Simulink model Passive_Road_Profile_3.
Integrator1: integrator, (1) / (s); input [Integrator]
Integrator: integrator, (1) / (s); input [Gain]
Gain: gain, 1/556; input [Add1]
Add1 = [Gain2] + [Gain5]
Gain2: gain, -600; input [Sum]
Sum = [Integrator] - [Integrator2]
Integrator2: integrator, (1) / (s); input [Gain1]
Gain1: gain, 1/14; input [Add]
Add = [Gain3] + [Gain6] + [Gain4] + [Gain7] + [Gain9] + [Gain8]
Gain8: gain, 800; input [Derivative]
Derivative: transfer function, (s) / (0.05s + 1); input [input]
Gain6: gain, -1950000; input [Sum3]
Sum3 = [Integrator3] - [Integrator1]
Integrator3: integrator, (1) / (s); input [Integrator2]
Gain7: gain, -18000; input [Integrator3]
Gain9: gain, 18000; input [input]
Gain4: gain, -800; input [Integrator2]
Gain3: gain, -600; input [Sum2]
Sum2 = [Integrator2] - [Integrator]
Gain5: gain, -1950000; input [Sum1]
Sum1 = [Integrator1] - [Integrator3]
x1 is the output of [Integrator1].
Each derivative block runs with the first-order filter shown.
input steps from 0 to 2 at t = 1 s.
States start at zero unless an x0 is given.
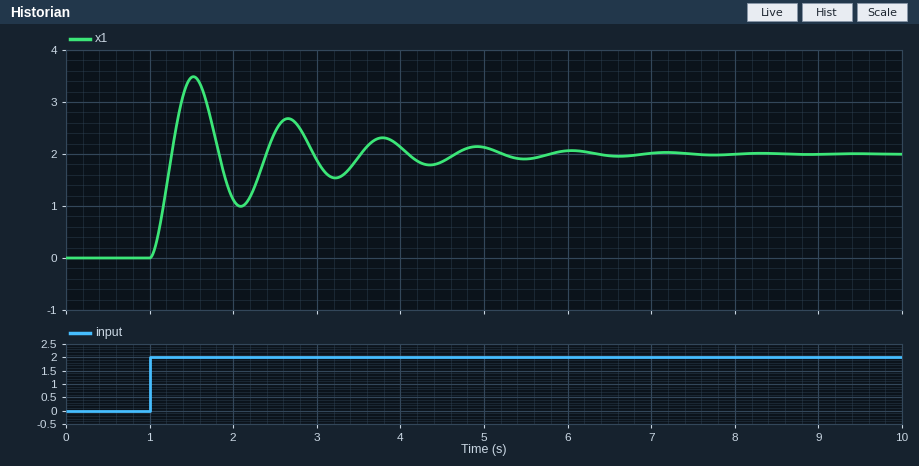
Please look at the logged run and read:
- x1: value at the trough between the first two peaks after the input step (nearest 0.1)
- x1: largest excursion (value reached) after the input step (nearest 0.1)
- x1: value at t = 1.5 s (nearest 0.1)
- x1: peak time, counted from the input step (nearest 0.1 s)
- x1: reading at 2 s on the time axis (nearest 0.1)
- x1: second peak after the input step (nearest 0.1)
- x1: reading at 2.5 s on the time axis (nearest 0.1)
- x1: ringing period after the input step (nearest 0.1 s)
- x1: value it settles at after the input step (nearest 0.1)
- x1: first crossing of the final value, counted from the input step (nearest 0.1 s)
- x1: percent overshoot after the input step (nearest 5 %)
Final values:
1.0
3.5
3.5
0.5 s
1.1
2.7
2.4
1.1 s
2.0
0.3 s
75 %
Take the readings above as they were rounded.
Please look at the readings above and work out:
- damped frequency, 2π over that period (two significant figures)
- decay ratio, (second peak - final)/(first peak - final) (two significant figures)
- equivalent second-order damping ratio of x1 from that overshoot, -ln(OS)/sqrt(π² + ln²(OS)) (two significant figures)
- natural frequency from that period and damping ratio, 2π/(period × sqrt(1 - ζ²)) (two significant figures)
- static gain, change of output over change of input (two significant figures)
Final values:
5.7 rad/s
0.47
0.091
5.7 rad/s
1.0
